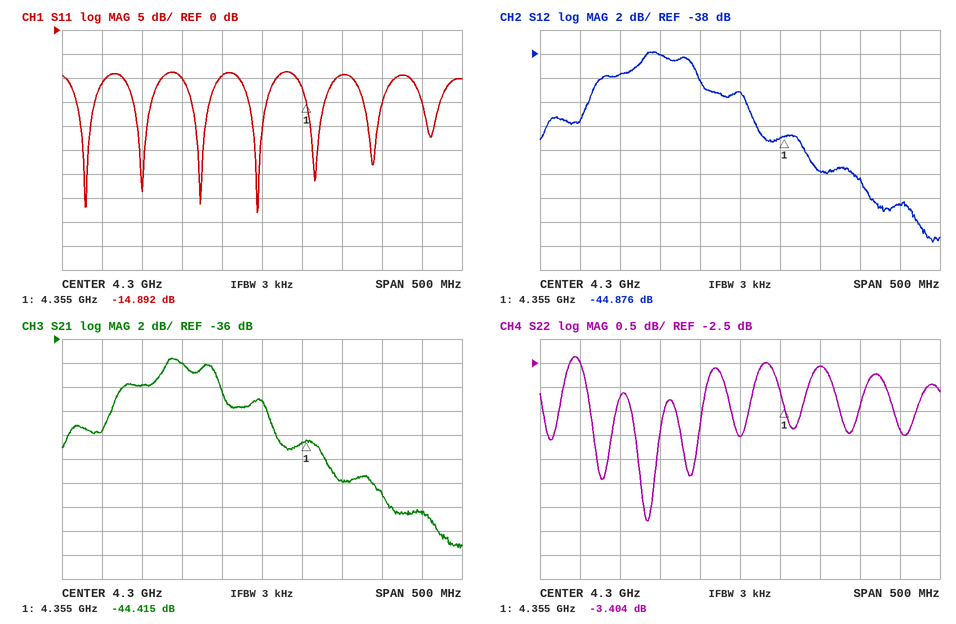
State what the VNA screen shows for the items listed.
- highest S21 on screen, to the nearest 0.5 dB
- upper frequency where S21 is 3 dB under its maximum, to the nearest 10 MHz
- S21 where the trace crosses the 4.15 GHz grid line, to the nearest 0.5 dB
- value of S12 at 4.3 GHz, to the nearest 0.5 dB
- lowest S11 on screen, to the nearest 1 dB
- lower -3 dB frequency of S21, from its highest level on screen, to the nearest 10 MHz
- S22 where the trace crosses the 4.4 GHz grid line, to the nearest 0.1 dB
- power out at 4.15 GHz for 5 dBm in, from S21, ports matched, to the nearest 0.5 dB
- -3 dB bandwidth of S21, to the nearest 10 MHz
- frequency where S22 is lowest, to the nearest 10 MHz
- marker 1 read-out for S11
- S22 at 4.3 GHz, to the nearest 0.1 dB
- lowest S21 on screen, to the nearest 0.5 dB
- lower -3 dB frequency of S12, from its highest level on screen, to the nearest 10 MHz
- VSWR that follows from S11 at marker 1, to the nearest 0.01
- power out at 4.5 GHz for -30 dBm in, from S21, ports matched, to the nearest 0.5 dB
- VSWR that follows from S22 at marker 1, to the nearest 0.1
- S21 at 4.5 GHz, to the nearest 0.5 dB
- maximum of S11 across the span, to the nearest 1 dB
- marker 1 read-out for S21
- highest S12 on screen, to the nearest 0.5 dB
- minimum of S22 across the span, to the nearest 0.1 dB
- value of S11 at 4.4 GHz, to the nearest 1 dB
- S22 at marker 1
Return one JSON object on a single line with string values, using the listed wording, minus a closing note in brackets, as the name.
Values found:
{"highest S21 on screen, to the nearest 0.5 dB": "-37.5 dB", "upper frequency where S21 is 3 dB under its maximum, to the nearest 10 MHz": "4.25 GHz", "S21 where the trace crosses the 4.15 GHz grid line, to the nearest 0.5 dB": "-40.0 dB", "value of S12 at 4.3 GHz, to the nearest 0.5 dB": "-41.0 dB", "lowest S11 on screen, to the nearest 1 dB": "-38 dB", "lower -3 dB frequency of S21, from its highest level on screen, to the nearest 10 MHz": "4.12 GHz", "S22 where the trace crosses the 4.4 GHz grid line, to the nearest 0.1 dB": "-2.6 dB", "power out at 4.15 GHz for 5 dBm in, from S21, ports matched, to the nearest 0.5 dB": "-35.0 dBm", "-3 dB bandwidth of S21, to the nearest 10 MHz": "130 MHz", "frequency where S22 is lowest, to the nearest 10 MHz": "4.18 GHz", "marker 1 read-out for S11": "-14.892 dB", "S22 at 4.3 GHz, to the nearest 0.1 dB": "-4.0 dB", "lowest S21 on screen, to the nearest 0.5 dB": "-53.5 dB", "lower -3 dB frequency of S12, from its highest level on screen, to the nearest 10 MHz": "4.12 GHz", "VSWR that follows from S11 at marker 1, to the nearest 0.01": "1.44", "power out at 4.5 GHz for -30 dBm in, from S21, ports matched, to the nearest 0.5 dB": "-80.5 dBm", "VSWR that follows from S22 at marker 1, to the nearest 0.1": "5.2", "S21 at 4.5 GHz, to the nearest 0.5 dB": "-50.5 dB", "maximum of S11 across the span, to the nearest 1 dB": "-9 dB", "marker 1 read-out for S21": "-44.415 dB", "highest S12 on screen, to the nearest 0.5 dB": "-38.0 dB", "minimum of S22 across the span, to the nearest 0.1 dB": "-5.8 dB", "value of S11 at 4.4 GHz, to the nearest 1 dB": "-9 dB", "S22 at marker 1": "-3.404 dB"}
